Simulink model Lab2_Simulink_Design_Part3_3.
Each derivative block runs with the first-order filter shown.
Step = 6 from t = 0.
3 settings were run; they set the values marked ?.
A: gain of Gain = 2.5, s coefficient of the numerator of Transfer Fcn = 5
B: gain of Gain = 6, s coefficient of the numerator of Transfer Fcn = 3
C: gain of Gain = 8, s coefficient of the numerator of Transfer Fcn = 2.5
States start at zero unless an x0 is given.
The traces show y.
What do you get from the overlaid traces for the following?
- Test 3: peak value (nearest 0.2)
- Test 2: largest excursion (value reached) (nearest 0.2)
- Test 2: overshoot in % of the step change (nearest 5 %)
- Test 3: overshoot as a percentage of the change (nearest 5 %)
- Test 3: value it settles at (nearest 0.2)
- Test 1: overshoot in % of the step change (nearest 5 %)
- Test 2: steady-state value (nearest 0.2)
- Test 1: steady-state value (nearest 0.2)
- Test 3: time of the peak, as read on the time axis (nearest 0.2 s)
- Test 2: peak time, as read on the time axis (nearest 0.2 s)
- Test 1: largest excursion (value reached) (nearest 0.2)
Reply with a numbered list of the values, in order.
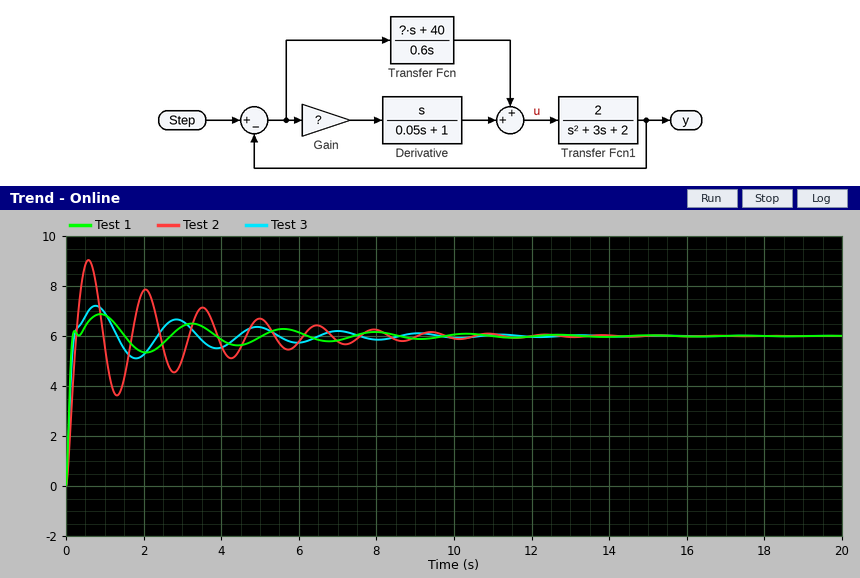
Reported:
1. 7.2
2. 9.0
3. 50 %
4. 20 %
5. 6.0
6. 15 %
7. 6.0
8. 6.0
9. 0.8 s
10. 0.6 s
11. 6.8
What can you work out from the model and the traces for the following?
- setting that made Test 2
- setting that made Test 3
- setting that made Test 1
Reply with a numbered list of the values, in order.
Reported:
1. A
2. B
3. C
